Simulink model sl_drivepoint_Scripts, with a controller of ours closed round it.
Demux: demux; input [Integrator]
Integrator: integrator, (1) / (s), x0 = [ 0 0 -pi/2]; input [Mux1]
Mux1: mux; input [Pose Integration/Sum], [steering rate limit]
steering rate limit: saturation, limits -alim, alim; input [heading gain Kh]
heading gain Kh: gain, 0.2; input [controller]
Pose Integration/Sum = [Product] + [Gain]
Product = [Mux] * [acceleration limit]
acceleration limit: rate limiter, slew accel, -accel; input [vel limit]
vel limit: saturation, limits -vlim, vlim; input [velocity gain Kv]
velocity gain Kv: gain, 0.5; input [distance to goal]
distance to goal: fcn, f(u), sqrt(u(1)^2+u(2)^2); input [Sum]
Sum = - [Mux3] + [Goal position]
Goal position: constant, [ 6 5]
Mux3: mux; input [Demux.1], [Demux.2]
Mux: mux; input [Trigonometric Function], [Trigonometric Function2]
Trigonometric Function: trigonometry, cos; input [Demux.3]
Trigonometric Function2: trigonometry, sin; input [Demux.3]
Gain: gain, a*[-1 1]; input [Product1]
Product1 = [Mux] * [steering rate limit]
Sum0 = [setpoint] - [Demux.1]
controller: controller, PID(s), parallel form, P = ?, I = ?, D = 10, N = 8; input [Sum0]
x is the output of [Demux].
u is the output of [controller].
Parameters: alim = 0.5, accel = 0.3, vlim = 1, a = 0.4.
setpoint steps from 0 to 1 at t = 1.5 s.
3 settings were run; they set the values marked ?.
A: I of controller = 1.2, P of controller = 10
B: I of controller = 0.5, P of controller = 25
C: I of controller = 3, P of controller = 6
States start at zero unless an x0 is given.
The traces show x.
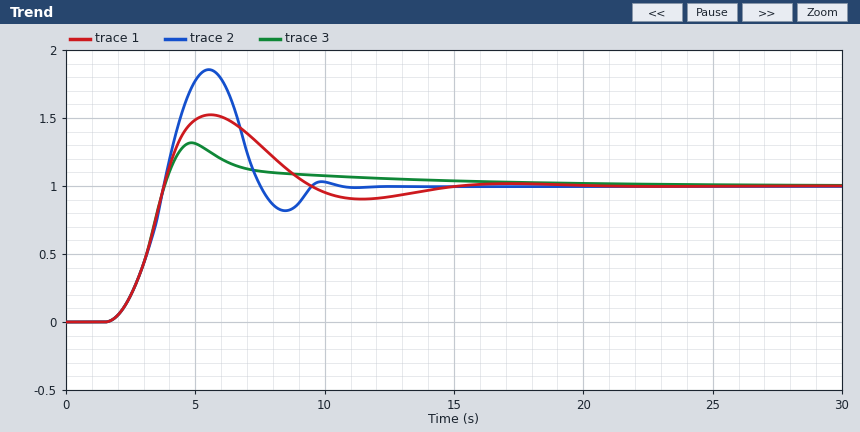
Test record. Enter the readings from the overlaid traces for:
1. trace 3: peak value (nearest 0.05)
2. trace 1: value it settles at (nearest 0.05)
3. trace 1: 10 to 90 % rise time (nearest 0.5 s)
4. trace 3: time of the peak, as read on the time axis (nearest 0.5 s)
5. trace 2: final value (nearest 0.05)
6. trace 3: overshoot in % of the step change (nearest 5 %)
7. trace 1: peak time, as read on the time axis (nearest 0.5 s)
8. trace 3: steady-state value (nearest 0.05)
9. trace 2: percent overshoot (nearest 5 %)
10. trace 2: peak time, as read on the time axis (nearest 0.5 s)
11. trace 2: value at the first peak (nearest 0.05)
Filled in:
1.30
1.00
1.5 s
5.0 s
1.00
30 %
5.5 s
1.00
85 %
5.5 s
1.85
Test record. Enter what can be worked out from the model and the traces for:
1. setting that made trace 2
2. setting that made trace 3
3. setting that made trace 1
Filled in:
B
A
C
